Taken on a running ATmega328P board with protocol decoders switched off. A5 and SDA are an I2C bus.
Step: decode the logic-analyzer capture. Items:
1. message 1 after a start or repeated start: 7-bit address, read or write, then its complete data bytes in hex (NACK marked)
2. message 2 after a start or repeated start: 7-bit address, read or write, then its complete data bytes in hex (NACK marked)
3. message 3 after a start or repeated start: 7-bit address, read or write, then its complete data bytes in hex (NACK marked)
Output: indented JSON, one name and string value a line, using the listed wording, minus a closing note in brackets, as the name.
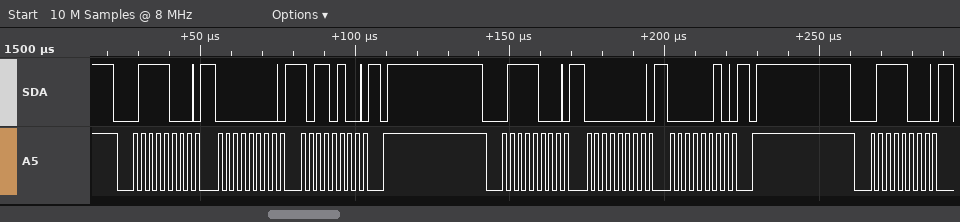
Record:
{
  "message 1 after a start or repeated start: 7-bit address, read or write, then its complete data bytes in hex": "0x3C write: 00 B4",
  "message 2 after a start or repeated start: 7-bit address, read or write, then its complete data bytes in hex": "0x3C write: 00 02",
  "message 3 after a start or repeated start: 7-bit address, read or write, then its complete data bytes in hex": "0x3C write"
}
